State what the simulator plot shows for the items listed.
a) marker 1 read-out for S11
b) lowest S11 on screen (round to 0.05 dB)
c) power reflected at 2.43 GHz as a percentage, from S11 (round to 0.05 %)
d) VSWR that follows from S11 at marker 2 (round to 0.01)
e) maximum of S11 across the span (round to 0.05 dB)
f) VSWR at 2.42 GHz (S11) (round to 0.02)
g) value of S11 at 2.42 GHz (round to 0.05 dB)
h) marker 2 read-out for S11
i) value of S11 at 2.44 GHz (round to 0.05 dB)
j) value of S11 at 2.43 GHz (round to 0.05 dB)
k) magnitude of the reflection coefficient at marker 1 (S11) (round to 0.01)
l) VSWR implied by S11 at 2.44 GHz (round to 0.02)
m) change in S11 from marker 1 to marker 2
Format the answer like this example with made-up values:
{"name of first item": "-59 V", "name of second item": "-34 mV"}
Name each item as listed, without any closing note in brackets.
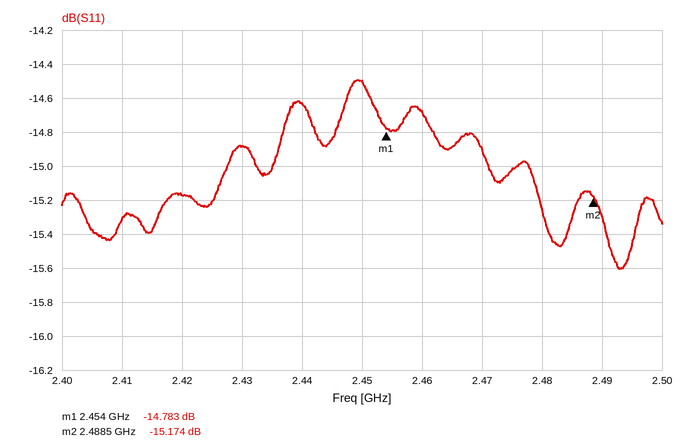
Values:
{"marker 1 read-out for S11": "-14.783 dB", "lowest S11 on screen": "-15.60 dB", "power reflected at 2.43 GHz as a percentage, from S11": "3.25 %", "VSWR that follows from S11 at marker 2": "1.42", "maximum of S11 across the span": "-14.50 dB", "VSWR at 2.42 GHz (S11)": "1.42", "value of S11 at 2.42 GHz": "-15.15 dB", "marker 2 read-out for S11": "-15.174 dB", "value of S11 at 2.44 GHz": "-14.65 dB", "value of S11 at 2.43 GHz": "-14.90 dB", "magnitude of the reflection coefficient at marker 1 (S11)": "0.18", "VSWR implied by S11 at 2.44 GHz": "1.46", "change in S11 from marker 1 to marker 2": "-0.391 dB"}
